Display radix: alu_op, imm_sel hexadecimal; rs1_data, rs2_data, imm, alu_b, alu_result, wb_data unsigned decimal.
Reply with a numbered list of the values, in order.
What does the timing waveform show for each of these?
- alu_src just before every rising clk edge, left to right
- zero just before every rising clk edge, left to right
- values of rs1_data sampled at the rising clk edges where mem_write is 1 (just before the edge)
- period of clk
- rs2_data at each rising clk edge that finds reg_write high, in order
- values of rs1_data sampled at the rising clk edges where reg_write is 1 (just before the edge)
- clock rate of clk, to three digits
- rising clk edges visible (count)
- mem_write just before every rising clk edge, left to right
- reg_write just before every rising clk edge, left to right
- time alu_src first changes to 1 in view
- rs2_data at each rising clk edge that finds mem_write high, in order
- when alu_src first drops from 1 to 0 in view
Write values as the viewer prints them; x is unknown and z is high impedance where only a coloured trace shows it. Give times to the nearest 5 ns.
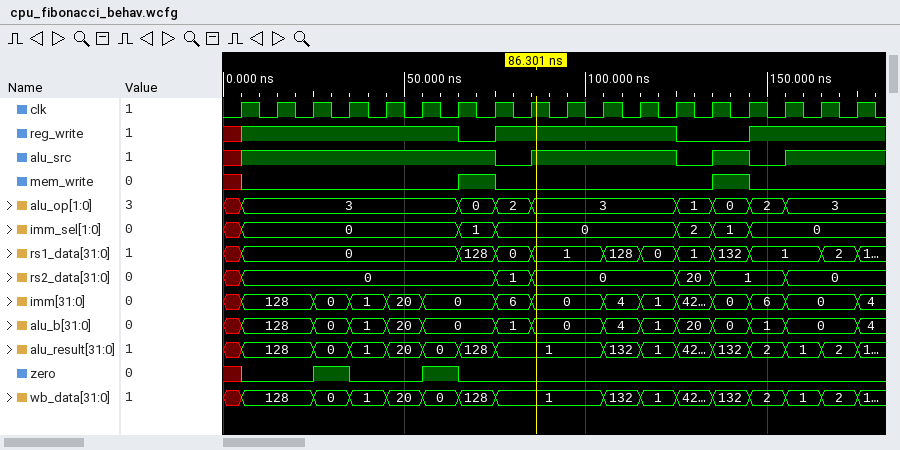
1. x 1 1 1 1 1 1 1 0 1 1 1 1 0 1 0 1 1
2. x 0 0 1 0 0 1 0 0 0 0 0 0 0 0 0 0 0
3. 128, 132
4. 10 ns
5. 0, 0, 0, 0, 0, 0, 1, 0, 0, 0, 0, 1, 0, 0
6. 0, 0, 0, 0, 0, 0, 0, 1, 1, 128, 0, 1, 1, 2
7. 100 MHz
8. 18
9. x 0 0 0 0 0 0 1 0 0 0 0 0 0 1 0 0 0
10. x 1 1 1 1 1 1 0 1 1 1 1 1 0 0 1 1 1
11. 5 ns
12. 0, 1
13. 75 ns
